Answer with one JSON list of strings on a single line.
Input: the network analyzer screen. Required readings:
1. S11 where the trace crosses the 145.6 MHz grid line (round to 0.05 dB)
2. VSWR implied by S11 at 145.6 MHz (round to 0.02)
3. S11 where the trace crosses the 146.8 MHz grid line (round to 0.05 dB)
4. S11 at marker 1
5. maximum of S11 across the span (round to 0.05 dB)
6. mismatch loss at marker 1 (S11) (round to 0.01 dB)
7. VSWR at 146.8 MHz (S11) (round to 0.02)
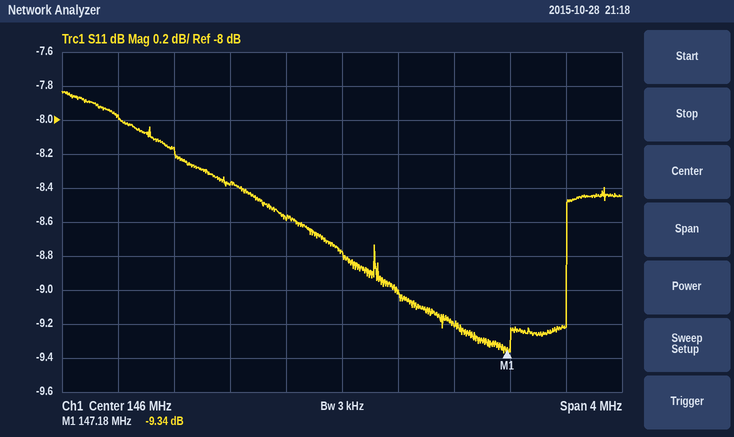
["-8.60 dB", "2.18", "-9.20 dB", "-9.34 dB", "-7.85 dB", "0.54 dB", "2.06"]
